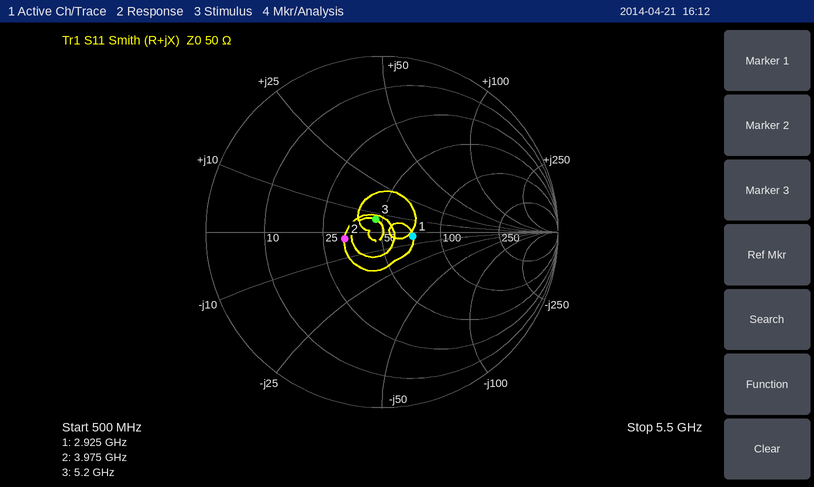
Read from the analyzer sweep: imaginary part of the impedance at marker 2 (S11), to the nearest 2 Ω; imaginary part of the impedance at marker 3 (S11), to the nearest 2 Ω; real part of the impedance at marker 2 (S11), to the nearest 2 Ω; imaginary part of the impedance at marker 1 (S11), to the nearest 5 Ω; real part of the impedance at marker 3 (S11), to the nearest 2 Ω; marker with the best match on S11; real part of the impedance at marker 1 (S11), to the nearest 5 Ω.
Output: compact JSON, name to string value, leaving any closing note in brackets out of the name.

{"imaginary part of the impedance at marker 2 (S11), to the nearest 2 Ω": "-2 Ω", "imaginary part of the impedance at marker 3 (S11), to the nearest 2 Ω": "+6 Ω", "real part of the impedance at marker 2 (S11), to the nearest 2 Ω": "32 Ω", "imaginary part of the impedance at marker 1 (S11), to the nearest 5 Ω": "-5 Ω", "real part of the impedance at marker 3 (S11), to the nearest 2 Ω": "46 Ω", "marker with the best match on S11": "marker 3", "real part of the impedance at marker 1 (S11), to the nearest 5 Ω": "70 Ω"}
